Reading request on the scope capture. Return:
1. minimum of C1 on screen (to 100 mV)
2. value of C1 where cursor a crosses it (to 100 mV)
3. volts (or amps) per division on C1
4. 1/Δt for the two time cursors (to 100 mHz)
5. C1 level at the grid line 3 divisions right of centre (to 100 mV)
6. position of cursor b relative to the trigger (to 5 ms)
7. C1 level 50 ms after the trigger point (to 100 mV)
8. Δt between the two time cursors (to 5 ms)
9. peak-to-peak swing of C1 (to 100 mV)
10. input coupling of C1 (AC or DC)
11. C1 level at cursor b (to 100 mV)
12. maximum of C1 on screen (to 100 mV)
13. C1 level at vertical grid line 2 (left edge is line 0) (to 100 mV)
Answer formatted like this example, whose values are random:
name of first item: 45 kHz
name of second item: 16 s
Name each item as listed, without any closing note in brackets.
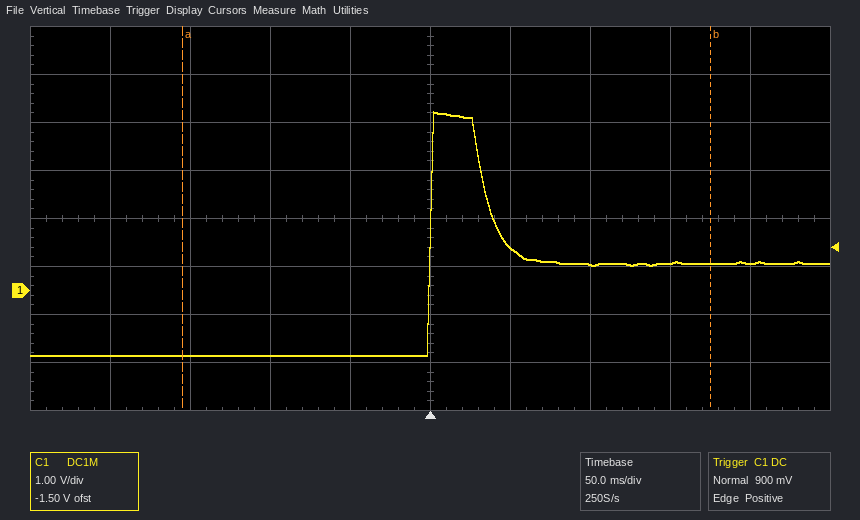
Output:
minimum of C1 on screen: -1.4 V
value of C1 where cursor a crosses it: -1.4 V
volts (or amps) per division on C1: 1 V
1/Δt for the two time cursors: 3.0 Hz
C1 level at the grid line 3 divisions right of centre: 600 mV
position of cursor b relative to the trigger: +175 ms
C1 level 50 ms after the trigger point: 900 mV
Δt between the two time cursors: 330 ms
peak-to-peak swing of C1: 5.1 V
input coupling of C1: DC
C1 level at cursor b: 600 mV
maximum of C1 on screen: 3.7 V
C1 level at vertical grid line 2 (left edge is line 0): -1.4 V
